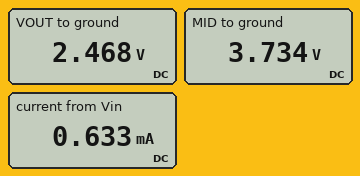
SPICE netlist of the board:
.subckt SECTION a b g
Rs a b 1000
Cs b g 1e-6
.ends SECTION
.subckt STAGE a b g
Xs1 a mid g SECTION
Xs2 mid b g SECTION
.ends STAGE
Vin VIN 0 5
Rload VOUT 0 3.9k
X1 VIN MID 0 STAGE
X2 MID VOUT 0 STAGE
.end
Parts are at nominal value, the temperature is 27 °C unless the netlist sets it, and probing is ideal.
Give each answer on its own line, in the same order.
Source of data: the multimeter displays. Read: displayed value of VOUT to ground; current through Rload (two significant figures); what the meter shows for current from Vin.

2.468 V
630 µA
0.633 mA
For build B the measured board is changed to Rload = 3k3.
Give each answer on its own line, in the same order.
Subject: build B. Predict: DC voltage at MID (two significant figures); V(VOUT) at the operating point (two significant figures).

3.6 V
2.3 V
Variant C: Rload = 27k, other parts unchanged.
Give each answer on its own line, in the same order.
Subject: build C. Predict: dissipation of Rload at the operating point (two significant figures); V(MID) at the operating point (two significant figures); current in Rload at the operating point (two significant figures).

700 µW
4.7 V
160 µA
